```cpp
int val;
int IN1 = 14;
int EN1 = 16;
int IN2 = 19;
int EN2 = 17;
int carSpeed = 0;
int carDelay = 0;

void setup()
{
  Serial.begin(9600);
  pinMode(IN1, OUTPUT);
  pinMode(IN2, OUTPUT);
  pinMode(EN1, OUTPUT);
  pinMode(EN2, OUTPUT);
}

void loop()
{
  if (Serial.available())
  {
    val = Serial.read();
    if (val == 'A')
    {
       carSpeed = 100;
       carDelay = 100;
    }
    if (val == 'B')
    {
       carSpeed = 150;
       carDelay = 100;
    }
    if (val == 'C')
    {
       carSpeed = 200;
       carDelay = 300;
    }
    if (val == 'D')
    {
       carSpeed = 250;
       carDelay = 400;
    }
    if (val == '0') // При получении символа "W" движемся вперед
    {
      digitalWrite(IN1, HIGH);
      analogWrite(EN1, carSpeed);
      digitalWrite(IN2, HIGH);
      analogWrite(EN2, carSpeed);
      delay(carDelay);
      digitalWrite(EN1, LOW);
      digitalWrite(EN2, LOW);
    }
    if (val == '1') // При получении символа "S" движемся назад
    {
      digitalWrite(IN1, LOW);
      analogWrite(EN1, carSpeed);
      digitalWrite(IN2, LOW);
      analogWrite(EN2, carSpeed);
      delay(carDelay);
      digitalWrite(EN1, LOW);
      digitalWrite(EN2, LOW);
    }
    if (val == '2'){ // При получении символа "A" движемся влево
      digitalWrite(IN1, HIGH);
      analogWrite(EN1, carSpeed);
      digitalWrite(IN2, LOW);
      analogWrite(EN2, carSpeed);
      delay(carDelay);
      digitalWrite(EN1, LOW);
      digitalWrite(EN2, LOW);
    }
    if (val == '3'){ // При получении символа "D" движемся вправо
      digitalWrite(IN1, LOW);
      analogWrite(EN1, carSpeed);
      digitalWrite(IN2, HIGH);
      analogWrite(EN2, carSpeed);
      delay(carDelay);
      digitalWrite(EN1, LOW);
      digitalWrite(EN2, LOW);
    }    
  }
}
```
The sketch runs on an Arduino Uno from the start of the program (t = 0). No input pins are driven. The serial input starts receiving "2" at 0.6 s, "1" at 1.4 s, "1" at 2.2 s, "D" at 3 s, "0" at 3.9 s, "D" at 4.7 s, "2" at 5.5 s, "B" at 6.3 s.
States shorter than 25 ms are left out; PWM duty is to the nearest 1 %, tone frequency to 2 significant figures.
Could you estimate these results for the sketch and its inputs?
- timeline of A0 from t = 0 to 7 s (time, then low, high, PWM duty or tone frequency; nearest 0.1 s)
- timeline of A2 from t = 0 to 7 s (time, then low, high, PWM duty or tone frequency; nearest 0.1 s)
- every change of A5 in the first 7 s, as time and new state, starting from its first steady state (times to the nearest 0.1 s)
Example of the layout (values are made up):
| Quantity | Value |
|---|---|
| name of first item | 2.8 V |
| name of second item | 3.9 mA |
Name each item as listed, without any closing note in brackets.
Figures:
| Quantity | Value |
|---|---|
| timeline of A0 from t = 0 to 7 s | 0 s low; 0.6 s high; 1.4 s low; 3.9 s high |
| timeline of A2 from t = 0 to 7 s | 0 s low; 3.9 s high; 4.3 s low; 5.5 s high; 5.9 s low |
| every change of A5 in the first 7 s, as time and new state, starting from its first steady state | 0 s low; 3.9 s high; 5.5 s low |
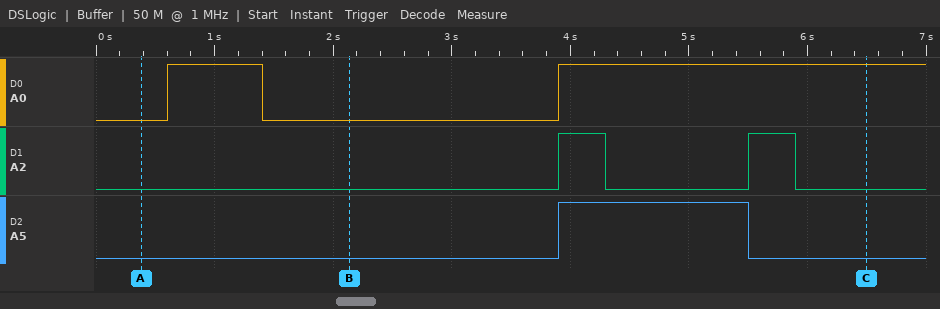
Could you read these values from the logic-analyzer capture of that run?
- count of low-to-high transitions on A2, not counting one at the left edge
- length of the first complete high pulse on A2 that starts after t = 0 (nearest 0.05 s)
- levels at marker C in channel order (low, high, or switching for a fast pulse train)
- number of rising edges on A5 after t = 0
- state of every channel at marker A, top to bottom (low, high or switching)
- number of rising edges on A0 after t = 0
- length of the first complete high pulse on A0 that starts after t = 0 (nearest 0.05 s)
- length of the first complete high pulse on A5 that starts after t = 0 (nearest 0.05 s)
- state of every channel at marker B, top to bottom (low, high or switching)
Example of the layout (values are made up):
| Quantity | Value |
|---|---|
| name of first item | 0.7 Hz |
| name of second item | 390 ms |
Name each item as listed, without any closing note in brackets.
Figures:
| Quantity | Value |
|---|---|
| count of low-to-high transitions on A2, not counting one at the left edge | 2 |
| length of the first complete high pulse on A2 that starts after t = 0 | 0.40 s |
| levels at marker C in channel order | A0 high, A2 low, A5 low |
| number of rising edges on A5 after t = 0 | 1 |
| state of every channel at marker A, top to bottom | A0 low, A2 low, A5 low |
| number of rising edges on A0 after t = 0 | 2 |
| length of the first complete high pulse on A0 that starts after t = 0 | 0.80 s |
| length of the first complete high pulse on A5 that starts after t = 0 | 1.60 s |
| state of every channel at marker B, top to bottom | A0 low, A2 low, A5 low |
